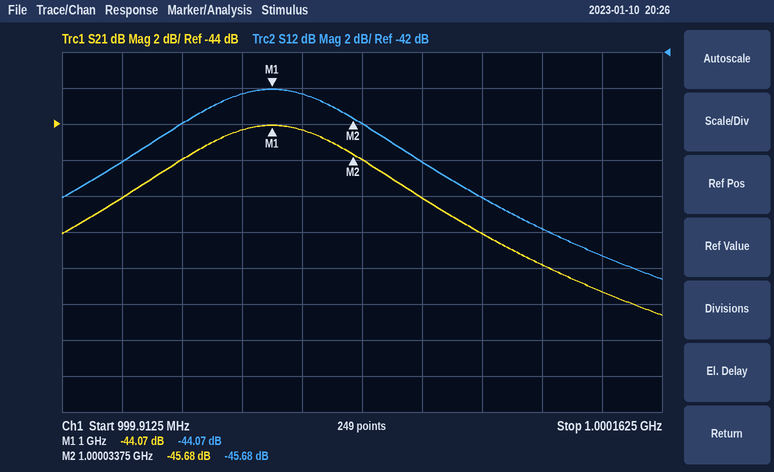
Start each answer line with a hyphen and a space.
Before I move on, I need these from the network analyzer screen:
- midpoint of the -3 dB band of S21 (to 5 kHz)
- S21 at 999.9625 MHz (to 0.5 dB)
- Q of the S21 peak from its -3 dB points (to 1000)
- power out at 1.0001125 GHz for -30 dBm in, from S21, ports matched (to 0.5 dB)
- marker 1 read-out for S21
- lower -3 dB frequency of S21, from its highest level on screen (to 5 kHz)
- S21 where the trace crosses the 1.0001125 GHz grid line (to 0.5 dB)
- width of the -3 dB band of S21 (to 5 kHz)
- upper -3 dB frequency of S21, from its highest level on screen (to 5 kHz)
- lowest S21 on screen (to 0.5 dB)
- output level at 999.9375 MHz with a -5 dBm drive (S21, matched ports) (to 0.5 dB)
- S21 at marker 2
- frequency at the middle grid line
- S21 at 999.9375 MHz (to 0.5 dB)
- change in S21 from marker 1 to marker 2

- 1.000000 GHz
- -46.0 dB
- 10000
- -82.0 dBm
- -44.07 dB
- 999.950 MHz
- -52.0 dB
- 100 kHz
- 1.000050 GHz
- -54.5 dB
- -53.0 dBm
- -45.68 dB
- 1.0000375 GHz
- -48.0 dB
- -1.61 dB
